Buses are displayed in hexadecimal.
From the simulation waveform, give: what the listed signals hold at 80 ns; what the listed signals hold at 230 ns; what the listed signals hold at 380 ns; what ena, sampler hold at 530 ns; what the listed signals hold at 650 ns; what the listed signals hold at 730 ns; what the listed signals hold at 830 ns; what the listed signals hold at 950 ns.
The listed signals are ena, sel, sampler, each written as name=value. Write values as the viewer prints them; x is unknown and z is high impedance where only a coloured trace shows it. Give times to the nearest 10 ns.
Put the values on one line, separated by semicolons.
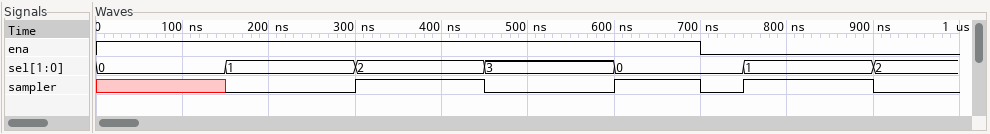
ena=1, sel=0, sampler=x; ena=1, sel=1, sampler=0; ena=1, sel=2, sampler=1; ena=1, sampler=0; ena=1, sel=0, sampler=1; ena=0, sel=0, sampler=0; ena=0, sel=1, sampler=1; ena=0, sel=2, sampler=0
